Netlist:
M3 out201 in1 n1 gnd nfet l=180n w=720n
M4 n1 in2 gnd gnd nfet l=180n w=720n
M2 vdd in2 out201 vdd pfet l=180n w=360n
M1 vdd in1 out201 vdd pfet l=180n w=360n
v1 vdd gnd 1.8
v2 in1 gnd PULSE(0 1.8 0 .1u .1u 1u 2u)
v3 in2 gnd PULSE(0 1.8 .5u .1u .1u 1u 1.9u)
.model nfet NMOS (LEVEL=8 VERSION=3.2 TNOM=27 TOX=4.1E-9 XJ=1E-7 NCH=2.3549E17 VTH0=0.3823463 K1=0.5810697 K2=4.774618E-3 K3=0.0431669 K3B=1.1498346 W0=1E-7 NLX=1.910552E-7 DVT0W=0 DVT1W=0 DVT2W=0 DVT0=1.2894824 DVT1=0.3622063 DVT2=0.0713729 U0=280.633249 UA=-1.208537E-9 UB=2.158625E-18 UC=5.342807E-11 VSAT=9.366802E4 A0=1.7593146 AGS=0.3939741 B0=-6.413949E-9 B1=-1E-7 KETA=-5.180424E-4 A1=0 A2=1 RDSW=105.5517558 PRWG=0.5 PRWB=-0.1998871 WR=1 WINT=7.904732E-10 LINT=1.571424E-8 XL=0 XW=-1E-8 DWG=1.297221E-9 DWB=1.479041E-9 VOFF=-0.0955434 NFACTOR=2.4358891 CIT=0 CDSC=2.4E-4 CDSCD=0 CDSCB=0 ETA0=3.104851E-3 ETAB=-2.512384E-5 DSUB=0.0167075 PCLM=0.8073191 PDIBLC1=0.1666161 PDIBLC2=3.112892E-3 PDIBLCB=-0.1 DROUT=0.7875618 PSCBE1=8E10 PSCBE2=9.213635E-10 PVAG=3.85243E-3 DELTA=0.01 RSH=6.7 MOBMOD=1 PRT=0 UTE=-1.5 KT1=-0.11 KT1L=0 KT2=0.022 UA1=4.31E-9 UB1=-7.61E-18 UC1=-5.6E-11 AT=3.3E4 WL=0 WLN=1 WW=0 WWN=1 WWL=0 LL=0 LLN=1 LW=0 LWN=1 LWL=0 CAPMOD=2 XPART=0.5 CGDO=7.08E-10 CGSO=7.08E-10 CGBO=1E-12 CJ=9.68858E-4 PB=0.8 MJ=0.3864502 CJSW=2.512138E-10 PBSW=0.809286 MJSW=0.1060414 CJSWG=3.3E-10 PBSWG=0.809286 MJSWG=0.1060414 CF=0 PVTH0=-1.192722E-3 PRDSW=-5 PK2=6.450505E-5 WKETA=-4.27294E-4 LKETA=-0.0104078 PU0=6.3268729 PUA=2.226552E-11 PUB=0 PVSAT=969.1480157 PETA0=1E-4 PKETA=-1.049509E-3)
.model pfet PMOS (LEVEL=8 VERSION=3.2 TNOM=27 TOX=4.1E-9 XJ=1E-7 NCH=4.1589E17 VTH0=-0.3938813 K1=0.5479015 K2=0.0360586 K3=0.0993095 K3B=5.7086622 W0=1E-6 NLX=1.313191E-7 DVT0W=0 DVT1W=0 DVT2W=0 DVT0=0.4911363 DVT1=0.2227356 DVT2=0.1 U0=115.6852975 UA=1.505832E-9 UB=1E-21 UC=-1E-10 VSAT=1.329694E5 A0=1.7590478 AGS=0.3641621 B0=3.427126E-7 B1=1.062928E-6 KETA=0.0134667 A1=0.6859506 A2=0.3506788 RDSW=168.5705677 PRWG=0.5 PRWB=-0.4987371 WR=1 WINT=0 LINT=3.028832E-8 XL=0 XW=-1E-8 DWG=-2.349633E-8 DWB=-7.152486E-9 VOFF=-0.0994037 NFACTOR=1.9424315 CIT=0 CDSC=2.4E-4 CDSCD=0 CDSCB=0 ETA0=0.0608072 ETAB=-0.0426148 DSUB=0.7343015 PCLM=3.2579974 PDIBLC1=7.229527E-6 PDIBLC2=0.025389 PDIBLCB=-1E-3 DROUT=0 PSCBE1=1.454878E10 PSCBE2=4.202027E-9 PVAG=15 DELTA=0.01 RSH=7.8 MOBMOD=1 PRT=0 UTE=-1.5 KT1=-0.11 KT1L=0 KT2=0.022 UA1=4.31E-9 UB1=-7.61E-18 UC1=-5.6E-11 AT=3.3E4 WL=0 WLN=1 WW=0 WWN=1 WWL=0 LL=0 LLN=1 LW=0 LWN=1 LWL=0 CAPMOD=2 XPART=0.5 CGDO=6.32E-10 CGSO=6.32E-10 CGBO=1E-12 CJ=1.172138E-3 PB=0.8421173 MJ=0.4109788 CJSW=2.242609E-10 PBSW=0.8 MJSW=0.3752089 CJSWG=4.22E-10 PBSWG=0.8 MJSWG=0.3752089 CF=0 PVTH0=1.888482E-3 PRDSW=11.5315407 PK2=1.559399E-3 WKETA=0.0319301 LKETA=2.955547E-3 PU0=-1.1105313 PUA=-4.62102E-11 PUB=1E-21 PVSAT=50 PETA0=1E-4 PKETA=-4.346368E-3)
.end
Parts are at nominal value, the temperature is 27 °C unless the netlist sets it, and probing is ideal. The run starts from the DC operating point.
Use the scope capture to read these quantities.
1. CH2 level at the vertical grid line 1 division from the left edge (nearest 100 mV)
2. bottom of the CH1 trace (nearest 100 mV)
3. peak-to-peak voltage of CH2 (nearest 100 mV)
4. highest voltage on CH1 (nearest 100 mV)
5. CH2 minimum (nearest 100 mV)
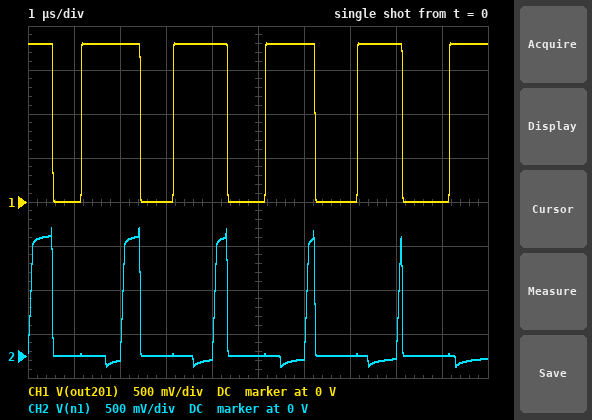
0 V
0 V
1.6 V
1.8 V
-100 mV
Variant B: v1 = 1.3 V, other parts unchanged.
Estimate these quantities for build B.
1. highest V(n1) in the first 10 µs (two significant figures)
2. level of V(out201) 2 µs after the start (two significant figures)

1.4 V
1.3 V
